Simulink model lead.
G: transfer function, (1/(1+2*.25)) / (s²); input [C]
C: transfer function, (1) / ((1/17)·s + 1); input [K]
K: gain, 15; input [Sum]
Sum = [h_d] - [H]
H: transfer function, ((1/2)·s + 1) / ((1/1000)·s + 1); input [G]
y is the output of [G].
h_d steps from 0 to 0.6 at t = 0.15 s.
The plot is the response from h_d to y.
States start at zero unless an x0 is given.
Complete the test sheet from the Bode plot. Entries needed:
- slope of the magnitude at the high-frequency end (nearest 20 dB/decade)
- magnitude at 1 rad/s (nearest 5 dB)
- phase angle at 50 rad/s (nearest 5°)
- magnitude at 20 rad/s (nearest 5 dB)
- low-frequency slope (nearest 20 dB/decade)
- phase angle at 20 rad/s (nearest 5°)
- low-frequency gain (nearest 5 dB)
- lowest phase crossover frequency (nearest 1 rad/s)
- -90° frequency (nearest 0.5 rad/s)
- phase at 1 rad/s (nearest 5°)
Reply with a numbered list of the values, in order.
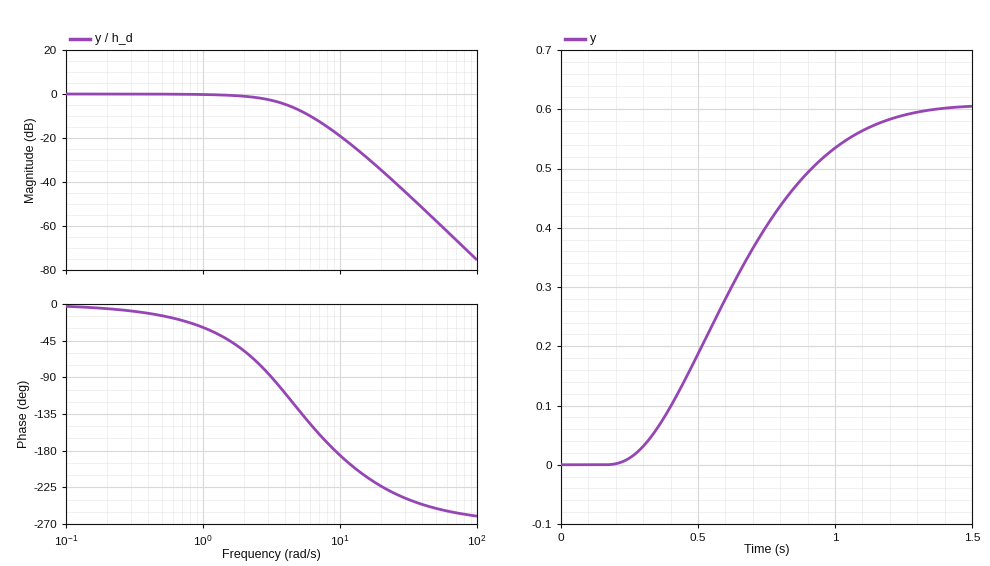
1. -60 dB/decade
2. 0 dB
3. -250°
4. -35 dB
5. 0 dB/decade
6. -225°
7. 0 dB
8. 9 rad/s
9. 3.0 rad/s
10. -30°
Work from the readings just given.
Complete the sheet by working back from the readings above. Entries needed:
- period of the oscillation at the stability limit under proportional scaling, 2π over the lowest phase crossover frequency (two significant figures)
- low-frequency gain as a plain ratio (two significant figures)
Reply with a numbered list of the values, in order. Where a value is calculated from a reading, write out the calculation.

1. 2π / 9 = 0.70 s
2. 10^(0 / 20) = 1.0
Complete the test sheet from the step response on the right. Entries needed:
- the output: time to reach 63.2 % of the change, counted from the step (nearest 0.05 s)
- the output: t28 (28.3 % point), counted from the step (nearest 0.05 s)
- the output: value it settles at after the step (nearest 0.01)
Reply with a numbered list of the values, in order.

1. 0.55 s
2. 0.35 s
3. 0.60
